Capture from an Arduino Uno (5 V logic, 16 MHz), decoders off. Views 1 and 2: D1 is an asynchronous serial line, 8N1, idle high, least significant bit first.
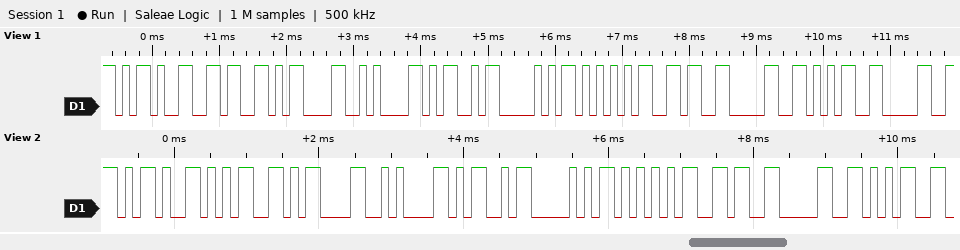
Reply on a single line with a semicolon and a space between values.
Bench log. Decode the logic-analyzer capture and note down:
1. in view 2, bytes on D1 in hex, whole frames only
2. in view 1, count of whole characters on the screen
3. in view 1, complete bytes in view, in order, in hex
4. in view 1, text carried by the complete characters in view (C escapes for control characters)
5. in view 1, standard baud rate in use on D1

2D 35 0D 0A 4D 50 55 36 30 35; 11; 2D 36 0D 0A 4D 50 55 36 30 35 30; "-6\r\nMPU6050"; 9600 baud
